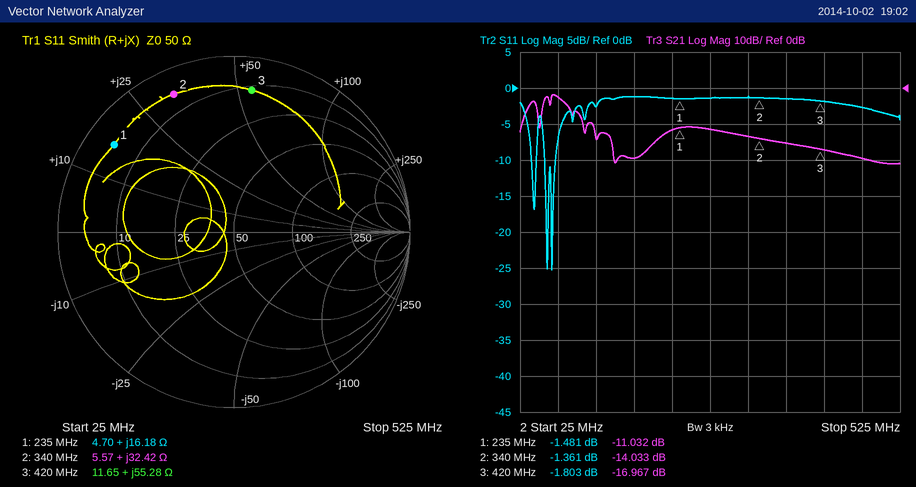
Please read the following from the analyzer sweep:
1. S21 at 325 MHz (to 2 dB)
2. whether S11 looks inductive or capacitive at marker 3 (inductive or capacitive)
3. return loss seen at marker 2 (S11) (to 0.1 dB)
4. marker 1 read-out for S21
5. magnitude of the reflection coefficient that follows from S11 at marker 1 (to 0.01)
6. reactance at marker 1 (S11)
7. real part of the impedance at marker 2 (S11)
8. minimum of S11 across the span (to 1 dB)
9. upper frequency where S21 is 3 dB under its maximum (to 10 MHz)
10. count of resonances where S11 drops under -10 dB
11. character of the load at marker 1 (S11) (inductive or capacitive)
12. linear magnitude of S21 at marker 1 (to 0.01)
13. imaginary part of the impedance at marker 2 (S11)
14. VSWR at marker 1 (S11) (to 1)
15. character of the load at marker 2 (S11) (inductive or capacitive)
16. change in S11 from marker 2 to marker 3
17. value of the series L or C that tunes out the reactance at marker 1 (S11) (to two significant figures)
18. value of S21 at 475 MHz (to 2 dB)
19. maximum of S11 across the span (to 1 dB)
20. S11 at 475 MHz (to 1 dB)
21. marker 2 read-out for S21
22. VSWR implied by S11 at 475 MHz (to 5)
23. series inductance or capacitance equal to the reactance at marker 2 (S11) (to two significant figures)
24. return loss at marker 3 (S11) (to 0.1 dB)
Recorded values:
-14 dB
inductive
1.4 dB
-11.032 dB
0.84
+16.18 Ω
5.57 Ω
-25 dB
90 MHz
3
inductive
0.28
+32.42 Ω
12
inductive
-0.442 dB
42 pF
-20 dB
-1 dB
-3 dB
-14.033 dB
5
15 nH
1.8 dB
